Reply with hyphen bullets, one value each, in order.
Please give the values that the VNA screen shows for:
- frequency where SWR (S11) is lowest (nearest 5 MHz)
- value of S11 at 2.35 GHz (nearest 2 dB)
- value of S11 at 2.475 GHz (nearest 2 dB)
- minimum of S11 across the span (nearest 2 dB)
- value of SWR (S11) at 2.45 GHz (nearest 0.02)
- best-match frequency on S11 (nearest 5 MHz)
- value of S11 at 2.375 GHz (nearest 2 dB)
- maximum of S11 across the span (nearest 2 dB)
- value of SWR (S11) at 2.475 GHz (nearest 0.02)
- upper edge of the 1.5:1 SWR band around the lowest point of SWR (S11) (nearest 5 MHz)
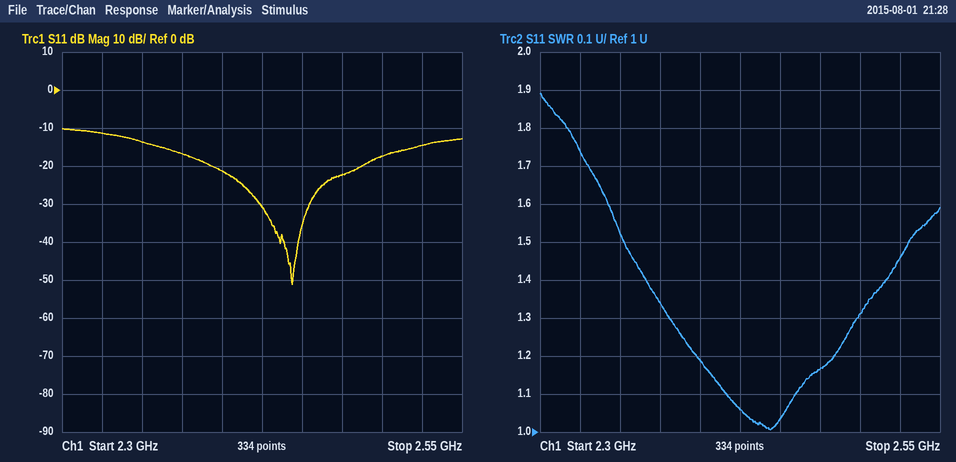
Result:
- 2.445 GHz
- -14 dB
- -22 dB
- -52 dB
- 1.04
- 2.445 GHz
- -16 dB
- -10 dB
- 1.16
- 2.530 GHz
